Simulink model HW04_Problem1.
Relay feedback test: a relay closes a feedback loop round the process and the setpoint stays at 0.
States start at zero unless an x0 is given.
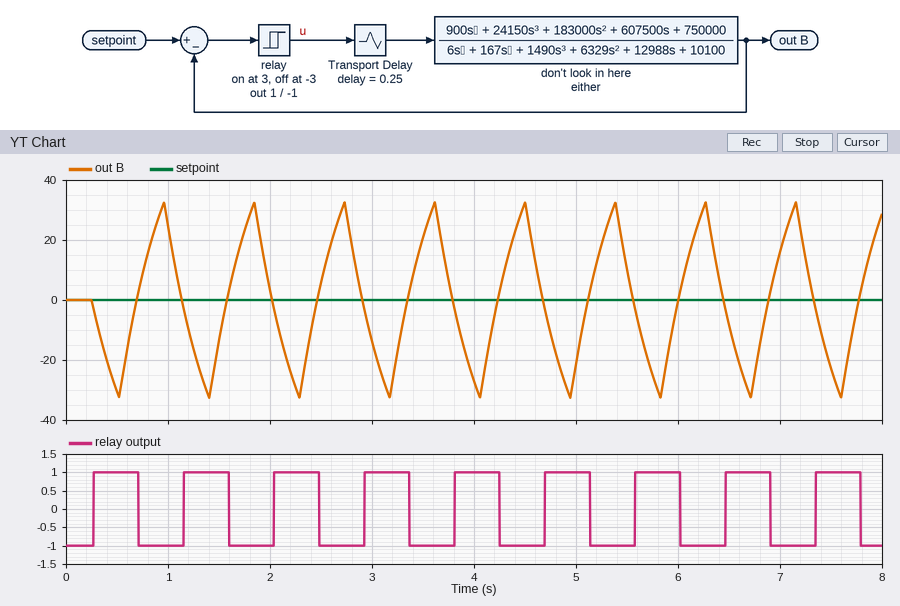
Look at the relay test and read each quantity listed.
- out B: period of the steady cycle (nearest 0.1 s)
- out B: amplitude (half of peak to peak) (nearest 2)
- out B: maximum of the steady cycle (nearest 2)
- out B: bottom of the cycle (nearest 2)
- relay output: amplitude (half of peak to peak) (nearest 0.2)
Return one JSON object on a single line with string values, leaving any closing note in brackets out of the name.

{"out B: period of the steady cycle": "0.9 s", "out B: amplitude (half of peak to peak)": "32", "out B: maximum of the steady cycle": "32", "out B: bottom of the cycle": "-32", "relay output: amplitude (half of peak to peak)": "1.0"}
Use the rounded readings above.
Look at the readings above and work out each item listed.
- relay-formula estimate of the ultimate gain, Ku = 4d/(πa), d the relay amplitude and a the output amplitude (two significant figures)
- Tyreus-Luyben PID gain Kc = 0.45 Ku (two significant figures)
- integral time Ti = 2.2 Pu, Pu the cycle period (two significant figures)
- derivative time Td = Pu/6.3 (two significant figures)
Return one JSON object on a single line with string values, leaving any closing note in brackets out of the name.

{"relay-formula estimate of the ultimate gain, Ku = 4d/(πa), d the relay amplitude and a the output amplitude": "0.040", "Tyreus-Luyben PID gain Kc = 0.45 Ku": "0.018", "integral time Ti = 2.2 Pu, Pu the cycle period": "2.0 s", "derivative time Td = Pu/6.3": "0.14 s"}
